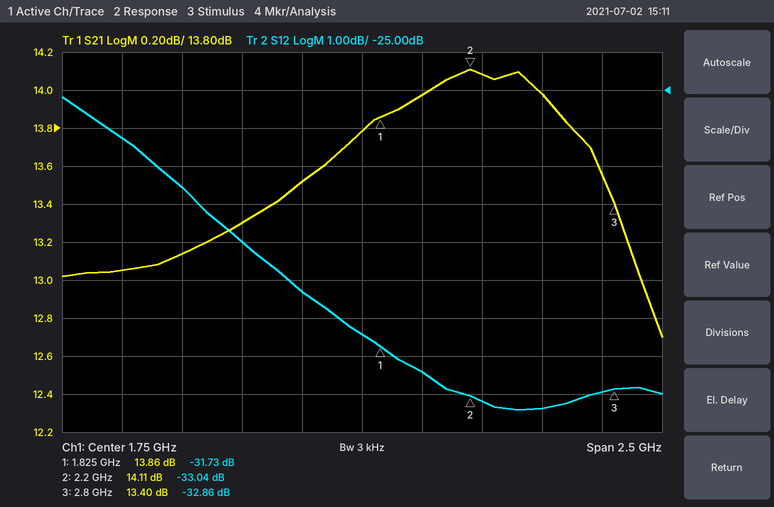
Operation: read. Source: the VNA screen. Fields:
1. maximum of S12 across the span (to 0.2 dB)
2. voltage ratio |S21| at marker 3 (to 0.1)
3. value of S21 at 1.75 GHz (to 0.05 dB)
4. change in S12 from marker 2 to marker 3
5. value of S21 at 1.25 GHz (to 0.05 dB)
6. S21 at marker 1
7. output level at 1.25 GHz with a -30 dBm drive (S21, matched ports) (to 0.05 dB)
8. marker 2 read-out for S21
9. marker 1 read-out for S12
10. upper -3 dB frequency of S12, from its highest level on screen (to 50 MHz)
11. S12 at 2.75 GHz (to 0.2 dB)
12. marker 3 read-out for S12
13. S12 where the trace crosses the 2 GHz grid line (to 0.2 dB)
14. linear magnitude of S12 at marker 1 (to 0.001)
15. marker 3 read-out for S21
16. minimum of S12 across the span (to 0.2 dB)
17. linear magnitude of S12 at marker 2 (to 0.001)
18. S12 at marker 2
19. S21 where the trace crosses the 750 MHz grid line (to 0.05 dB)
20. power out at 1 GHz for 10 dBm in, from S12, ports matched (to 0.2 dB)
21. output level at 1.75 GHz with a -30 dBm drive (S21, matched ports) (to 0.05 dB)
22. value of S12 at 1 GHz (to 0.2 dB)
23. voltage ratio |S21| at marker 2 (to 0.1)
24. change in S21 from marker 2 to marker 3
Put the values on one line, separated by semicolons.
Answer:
-25.2 dB; 4.7; 13.80 dB; 0.18 dB; 13.30 dB; 13.86 dB; -16.70 dBm; 14.11 dB; -31.73 dB; 1.10 GHz; -33.0 dB; -32.86 dB; -32.4 dB; 0.026; 13.40 dB; -33.4 dB; 0.022; -33.04 dB; 13.05 dB; -17.6 dBm; -16.20 dBm; -27.6 dB; 5.1; -0.71 dB
